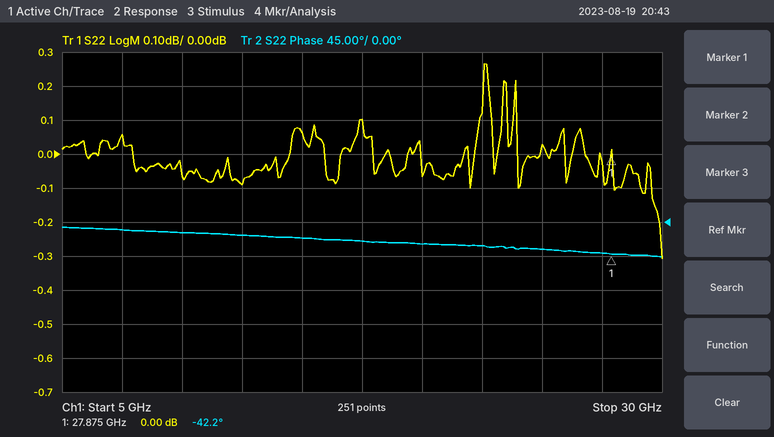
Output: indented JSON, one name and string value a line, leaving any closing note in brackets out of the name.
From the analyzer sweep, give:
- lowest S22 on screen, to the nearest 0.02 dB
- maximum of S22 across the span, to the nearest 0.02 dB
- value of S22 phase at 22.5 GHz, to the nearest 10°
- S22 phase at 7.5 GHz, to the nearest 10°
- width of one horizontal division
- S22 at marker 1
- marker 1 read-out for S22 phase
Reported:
{
  "lowest S22 on screen, to the nearest 0.02 dB": "-0.30 dB",
  "maximum of S22 across the span, to the nearest 0.02 dB": "0.26 dB",
  "value of S22 phase at 22.5 GHz, to the nearest 10°": "-30°",
  "S22 phase at 7.5 GHz, to the nearest 10°": "-10°",
  "width of one horizontal division": "2.5 GHz",
  "S22 at marker 1": "0.00 dB",
  "marker 1 read-out for S22 phase": "-42.2°"
}
